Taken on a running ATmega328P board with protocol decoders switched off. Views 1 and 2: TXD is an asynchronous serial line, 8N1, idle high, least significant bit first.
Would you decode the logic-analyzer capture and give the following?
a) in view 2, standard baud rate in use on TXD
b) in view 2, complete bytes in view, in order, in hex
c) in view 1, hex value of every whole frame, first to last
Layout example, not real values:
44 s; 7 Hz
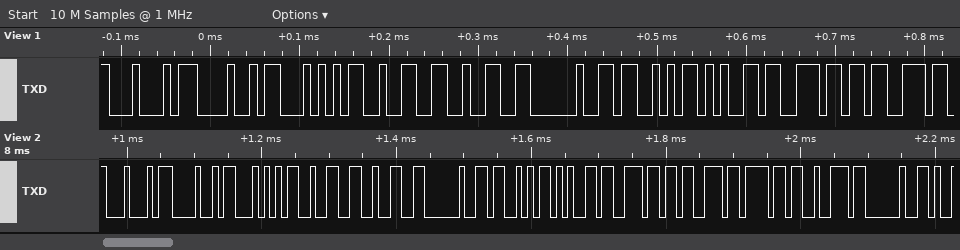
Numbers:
115200 baud; 44 48 54 32 32 20 53 65 6E 73 6F 72 20; 44 48 54 32 32 20 53 65 6E 73
